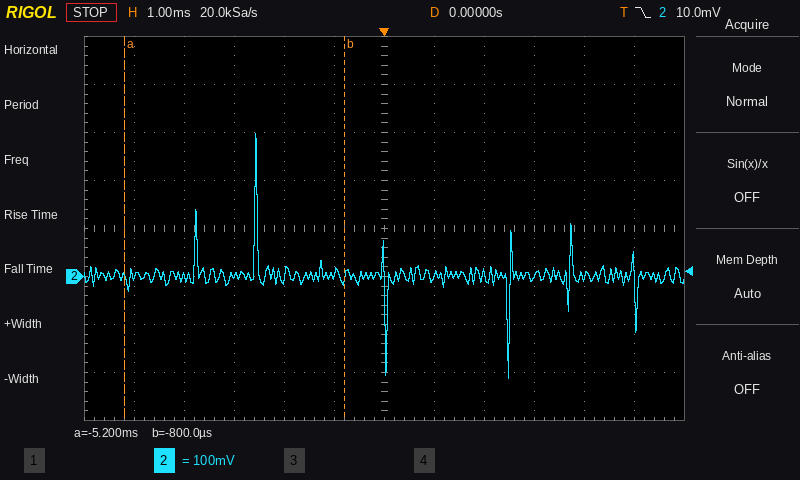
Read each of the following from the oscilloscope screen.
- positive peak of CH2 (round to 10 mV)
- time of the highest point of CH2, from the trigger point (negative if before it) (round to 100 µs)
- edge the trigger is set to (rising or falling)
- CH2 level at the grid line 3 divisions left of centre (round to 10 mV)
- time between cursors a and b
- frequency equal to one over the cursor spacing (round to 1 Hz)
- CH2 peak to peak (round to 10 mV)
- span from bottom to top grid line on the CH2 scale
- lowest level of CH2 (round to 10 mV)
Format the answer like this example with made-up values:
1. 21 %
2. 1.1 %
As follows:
1. 300 mV
2. -2.6 ms
3. falling
4. 0 mV
5. 4.4 ms
6. 227 Hz
7. 510 mV
8. 800 mV
9. -210 mV
